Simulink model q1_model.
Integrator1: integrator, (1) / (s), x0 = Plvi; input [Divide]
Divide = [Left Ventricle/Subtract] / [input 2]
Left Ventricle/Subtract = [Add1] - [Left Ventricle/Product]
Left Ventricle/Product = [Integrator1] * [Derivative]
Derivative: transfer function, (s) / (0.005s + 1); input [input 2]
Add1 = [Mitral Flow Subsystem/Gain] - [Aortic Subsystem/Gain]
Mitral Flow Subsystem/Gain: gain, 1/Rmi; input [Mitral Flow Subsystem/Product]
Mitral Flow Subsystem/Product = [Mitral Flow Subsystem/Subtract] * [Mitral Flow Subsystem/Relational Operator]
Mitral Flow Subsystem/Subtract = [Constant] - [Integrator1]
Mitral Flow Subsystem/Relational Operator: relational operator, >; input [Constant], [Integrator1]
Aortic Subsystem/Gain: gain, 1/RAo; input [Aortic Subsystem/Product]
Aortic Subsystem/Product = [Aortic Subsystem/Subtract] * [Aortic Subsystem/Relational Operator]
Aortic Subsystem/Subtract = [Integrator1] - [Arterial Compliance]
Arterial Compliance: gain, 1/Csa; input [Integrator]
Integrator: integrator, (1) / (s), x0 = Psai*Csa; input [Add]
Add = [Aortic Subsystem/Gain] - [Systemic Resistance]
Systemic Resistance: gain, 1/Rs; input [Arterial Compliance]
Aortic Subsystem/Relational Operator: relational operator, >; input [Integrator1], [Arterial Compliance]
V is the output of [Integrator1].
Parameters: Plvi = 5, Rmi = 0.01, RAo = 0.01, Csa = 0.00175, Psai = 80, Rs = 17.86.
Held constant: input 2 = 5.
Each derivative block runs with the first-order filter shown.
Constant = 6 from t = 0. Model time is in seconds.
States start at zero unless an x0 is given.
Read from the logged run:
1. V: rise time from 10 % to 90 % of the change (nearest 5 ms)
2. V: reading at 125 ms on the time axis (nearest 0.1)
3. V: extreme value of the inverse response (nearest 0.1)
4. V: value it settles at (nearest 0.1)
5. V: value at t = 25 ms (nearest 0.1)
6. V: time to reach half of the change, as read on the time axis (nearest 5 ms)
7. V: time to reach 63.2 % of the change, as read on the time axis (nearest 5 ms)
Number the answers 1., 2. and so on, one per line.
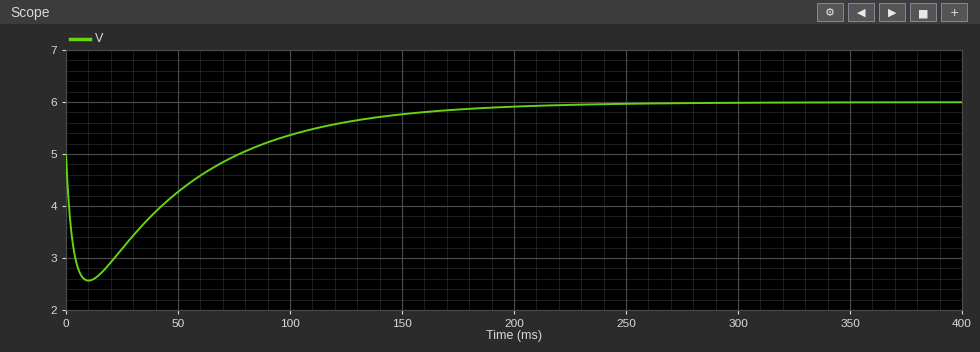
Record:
1. 110 ms
2. 5.6
3. 2.6
4. 6.0
5. 3.2
6. 110 ms
7. 125 ms
